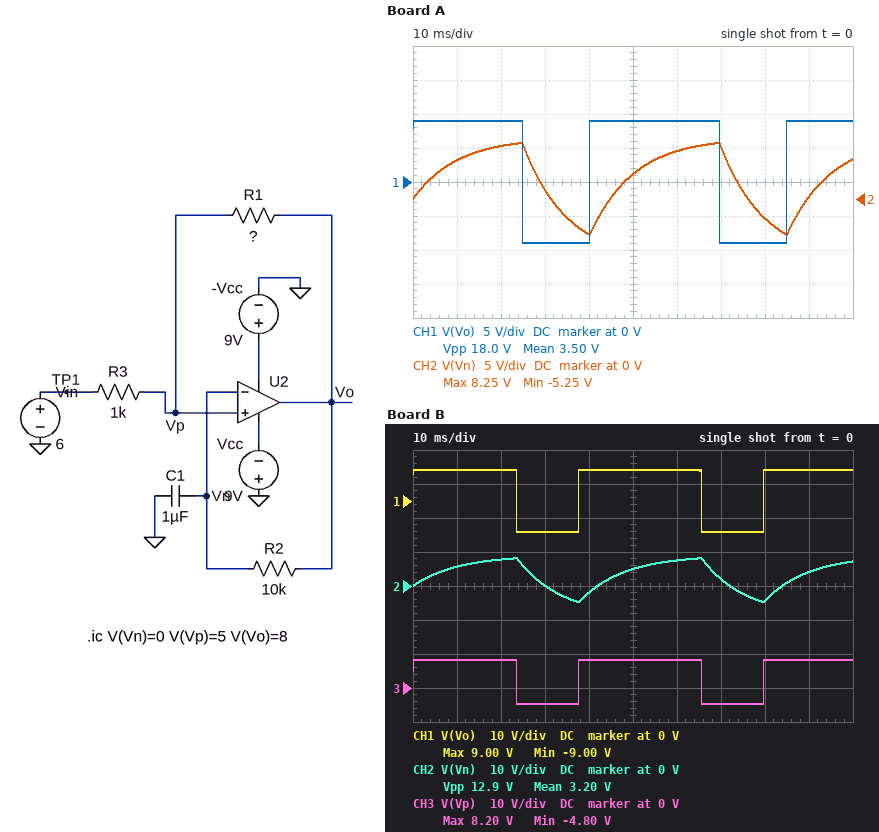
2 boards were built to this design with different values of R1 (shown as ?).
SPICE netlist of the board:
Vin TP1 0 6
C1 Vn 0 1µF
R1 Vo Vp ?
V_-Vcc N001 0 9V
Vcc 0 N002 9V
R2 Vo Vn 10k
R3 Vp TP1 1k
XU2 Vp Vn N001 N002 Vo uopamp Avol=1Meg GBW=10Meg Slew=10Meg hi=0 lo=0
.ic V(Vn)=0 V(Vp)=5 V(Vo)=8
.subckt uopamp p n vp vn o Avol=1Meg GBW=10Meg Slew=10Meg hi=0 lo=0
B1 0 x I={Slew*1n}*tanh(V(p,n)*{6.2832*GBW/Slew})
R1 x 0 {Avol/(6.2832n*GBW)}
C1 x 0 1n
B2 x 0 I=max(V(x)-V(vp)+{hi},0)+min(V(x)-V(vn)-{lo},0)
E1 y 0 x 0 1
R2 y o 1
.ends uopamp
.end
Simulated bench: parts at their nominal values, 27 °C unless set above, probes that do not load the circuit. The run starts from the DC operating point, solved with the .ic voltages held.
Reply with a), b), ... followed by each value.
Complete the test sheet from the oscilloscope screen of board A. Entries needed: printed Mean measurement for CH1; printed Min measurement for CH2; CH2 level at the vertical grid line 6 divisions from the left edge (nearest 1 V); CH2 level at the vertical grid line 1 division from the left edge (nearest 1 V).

a) 3.50 V
b) -5.25 V
c) 7 V
d) 6 V
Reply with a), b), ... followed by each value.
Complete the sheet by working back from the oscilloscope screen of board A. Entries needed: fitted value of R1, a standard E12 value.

a) 330 Ω
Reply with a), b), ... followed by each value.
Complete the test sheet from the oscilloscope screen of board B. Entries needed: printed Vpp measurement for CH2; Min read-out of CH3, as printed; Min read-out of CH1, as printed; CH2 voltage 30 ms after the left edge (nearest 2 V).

a) 12.9 V
b) -4.80 V
c) -9.00 V
d) 0 V
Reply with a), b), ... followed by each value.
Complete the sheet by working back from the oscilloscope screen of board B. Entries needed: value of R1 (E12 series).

a) 390 Ω
